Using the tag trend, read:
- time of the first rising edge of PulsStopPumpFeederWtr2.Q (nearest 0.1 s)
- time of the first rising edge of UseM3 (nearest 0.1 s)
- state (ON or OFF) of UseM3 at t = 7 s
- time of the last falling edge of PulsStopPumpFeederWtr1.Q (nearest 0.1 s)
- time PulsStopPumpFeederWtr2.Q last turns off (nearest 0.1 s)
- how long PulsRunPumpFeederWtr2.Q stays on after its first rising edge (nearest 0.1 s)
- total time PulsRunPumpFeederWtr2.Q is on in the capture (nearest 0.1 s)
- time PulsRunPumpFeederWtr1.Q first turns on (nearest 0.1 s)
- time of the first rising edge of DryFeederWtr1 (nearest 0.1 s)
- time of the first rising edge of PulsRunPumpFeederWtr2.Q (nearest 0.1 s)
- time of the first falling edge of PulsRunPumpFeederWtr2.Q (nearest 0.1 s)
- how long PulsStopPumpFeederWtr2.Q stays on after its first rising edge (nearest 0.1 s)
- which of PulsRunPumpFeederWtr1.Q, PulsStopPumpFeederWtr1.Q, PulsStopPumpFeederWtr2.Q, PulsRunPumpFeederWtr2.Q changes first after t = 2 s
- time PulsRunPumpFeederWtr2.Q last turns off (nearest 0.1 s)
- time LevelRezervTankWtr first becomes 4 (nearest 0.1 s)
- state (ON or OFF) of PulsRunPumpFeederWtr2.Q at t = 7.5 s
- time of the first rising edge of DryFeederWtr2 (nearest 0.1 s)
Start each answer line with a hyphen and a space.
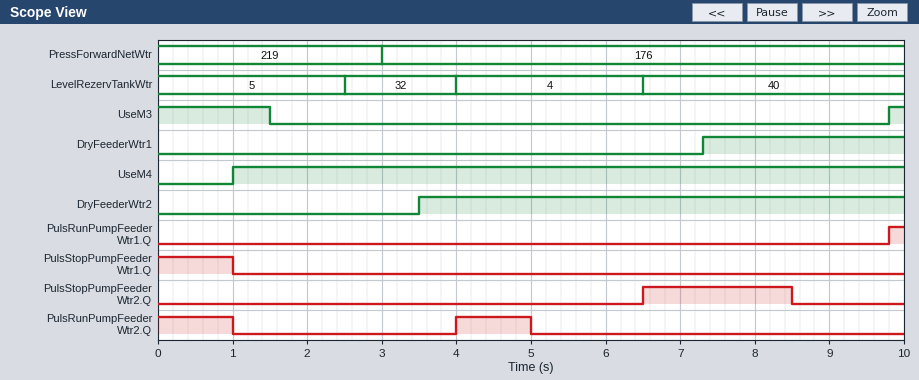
- 6.5 s
- 9.8 s
- OFF
- 1.0 s
- 8.5 s
- 1.0 s
- 2.0 s
- 9.8 s
- 7.3 s
- 4.0 s
- 1.0 s
- 2.0 s
- PulsRunPumpFeederWtr2.Q
- 5.0 s
- 4.0 s
- OFF
- 3.5 s
